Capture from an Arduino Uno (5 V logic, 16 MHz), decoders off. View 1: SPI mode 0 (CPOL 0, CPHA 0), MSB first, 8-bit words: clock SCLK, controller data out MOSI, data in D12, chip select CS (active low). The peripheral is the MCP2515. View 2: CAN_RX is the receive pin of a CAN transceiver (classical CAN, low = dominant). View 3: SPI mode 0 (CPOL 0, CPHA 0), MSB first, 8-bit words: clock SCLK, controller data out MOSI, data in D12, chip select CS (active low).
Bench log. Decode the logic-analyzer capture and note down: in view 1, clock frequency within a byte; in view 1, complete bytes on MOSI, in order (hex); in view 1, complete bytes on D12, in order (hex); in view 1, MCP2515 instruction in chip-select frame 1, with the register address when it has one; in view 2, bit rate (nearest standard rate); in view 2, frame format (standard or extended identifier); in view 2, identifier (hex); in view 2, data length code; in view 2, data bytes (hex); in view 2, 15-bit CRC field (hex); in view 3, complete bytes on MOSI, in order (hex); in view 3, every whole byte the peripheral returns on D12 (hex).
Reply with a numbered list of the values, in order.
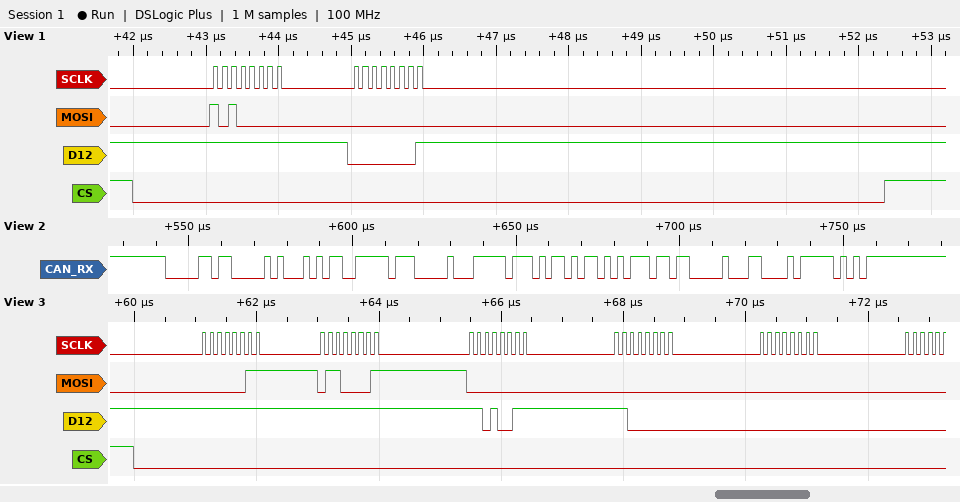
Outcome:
1. 8 MHz
2. 0xA0 0x00
3. 0xFF 0x01
4. READ STATUS
5. 500 kbit/s
6. standard
7. 0x058
8. 8
9. AC FF 00 FF 5A D5 DB 00
10. 0x617E
11. 0x03 0x61 0x00 0x00 0x00
12. 0xFF 0xFF 0xD3 0xC0 0x00
